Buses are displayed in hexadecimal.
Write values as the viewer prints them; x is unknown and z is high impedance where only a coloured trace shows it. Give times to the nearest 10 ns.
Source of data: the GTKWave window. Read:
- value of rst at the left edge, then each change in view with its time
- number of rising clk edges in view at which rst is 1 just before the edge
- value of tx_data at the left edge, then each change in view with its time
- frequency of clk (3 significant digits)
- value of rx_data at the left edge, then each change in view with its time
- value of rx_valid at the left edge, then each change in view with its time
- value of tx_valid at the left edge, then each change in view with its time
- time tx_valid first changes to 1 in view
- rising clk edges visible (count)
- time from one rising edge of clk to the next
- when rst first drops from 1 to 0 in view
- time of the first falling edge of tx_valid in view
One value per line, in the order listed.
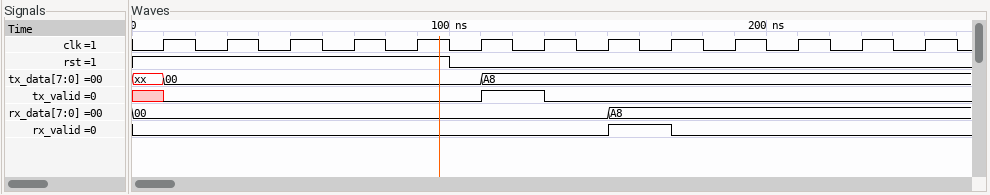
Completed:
1, 0 at 100 ns
5
xx, 00 at 10 ns, A8 at 110 ns
50.0 MHz
00, A8 at 150 ns
0, 1 at 150 ns, 0 at 170 ns
x, 0 at 10 ns, 1 at 110 ns, 0 at 130 ns
110 ns
13
20 ns
100 ns
130 ns
